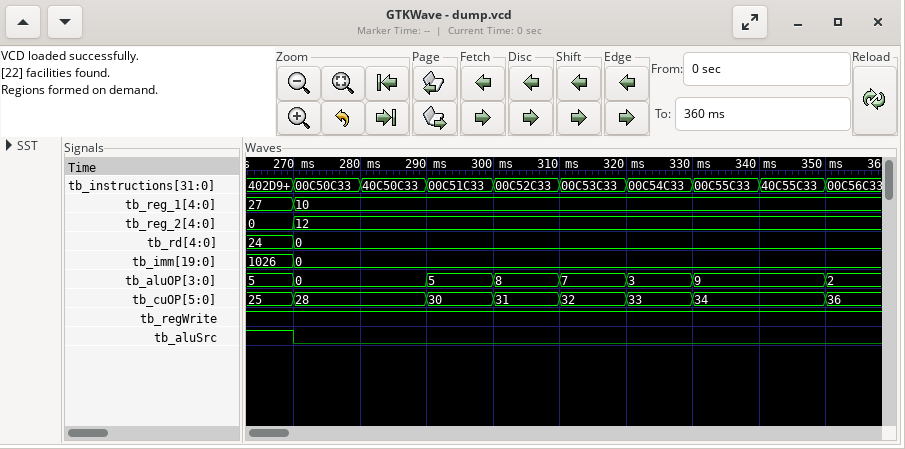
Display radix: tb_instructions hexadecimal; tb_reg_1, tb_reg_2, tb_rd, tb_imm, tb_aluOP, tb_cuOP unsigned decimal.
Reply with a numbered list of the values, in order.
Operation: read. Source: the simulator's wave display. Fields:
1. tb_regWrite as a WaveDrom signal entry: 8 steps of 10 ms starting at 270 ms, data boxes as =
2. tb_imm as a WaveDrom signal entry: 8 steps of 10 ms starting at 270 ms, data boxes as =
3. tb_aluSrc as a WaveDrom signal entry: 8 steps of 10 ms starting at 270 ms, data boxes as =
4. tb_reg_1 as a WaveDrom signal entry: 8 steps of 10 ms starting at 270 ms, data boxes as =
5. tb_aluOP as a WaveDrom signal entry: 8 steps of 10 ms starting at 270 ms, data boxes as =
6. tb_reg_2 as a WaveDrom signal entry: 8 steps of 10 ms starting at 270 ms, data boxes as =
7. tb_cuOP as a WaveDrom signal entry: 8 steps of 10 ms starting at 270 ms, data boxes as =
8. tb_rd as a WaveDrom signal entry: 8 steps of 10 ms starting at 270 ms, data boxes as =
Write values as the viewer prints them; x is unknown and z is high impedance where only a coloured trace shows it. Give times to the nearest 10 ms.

1. {name: 'tb_regWrite', wave: '1.......'}
2. {name: 'tb_imm', wave: '=.......', data: '0'}
3. {name: 'tb_aluSrc', wave: '0.......'}
4. {name: 'tb_reg_1', wave: '=.......', data: '10'}
5. {name: 'tb_aluOP', wave: '=.=====.', data: '0 5 8 7 3 9'}
6. {name: 'tb_reg_2', wave: '=.......', data: '12'}
7. {name: 'tb_cuOP', wave: '=.=====.', data: '28 30 31 32 33 34'}
8. {name: 'tb_rd', wave: '=.......', data: '0'}
